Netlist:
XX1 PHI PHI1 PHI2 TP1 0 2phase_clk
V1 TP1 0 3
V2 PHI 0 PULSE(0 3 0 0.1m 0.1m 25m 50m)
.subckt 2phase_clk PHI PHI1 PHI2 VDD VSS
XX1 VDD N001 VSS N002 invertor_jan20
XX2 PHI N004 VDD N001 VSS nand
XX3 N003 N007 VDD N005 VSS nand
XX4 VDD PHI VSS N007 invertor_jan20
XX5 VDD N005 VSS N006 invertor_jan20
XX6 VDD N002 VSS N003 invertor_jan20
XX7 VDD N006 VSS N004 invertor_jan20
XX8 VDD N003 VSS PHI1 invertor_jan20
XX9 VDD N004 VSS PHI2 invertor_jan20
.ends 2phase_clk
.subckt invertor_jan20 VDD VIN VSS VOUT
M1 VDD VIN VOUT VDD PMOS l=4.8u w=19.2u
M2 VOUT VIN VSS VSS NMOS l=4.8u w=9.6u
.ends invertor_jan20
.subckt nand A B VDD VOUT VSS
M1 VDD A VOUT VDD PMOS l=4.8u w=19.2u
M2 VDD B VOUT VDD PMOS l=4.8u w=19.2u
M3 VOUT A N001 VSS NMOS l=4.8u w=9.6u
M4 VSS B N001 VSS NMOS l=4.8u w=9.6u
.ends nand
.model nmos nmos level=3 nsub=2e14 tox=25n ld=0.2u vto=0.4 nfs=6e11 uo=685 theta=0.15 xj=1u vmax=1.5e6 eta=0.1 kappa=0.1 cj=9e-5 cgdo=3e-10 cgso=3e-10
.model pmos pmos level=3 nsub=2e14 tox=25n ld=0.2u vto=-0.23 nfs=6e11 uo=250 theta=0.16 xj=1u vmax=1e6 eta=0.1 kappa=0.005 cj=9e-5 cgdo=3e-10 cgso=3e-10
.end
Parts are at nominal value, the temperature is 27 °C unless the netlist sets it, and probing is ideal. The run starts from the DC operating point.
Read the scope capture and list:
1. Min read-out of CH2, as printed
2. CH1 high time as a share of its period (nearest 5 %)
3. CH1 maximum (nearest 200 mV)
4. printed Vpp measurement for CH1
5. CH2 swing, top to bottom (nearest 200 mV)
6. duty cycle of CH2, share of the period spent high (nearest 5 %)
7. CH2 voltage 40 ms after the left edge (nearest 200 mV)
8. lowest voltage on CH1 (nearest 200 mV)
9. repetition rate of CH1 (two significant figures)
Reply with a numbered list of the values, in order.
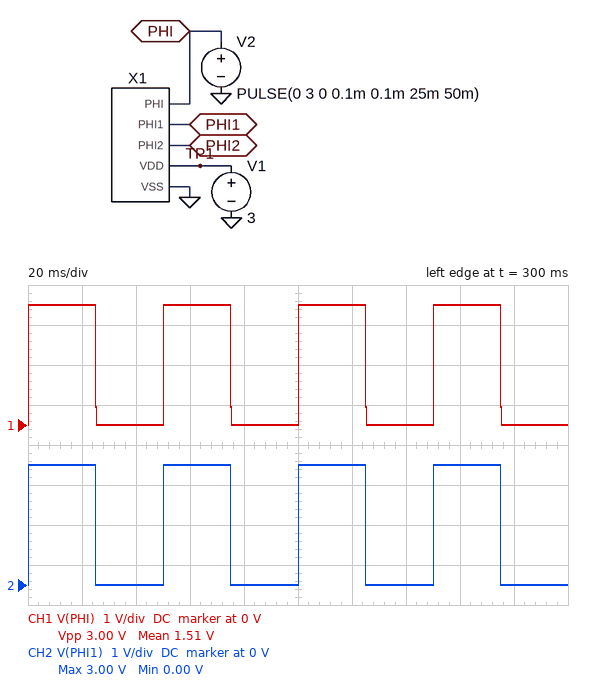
1. 0.00 V
2. 50 %
3. 3.0 V
4. 3.00 V
5. 3.0 V
6. 50 %
7. 0 V
8. 0 V
9. 20 Hz
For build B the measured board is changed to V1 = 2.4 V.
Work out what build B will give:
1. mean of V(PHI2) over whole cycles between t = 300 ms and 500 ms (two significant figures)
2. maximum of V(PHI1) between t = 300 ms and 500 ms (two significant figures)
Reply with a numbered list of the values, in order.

1. 1.2 V
2. 2.4 V
